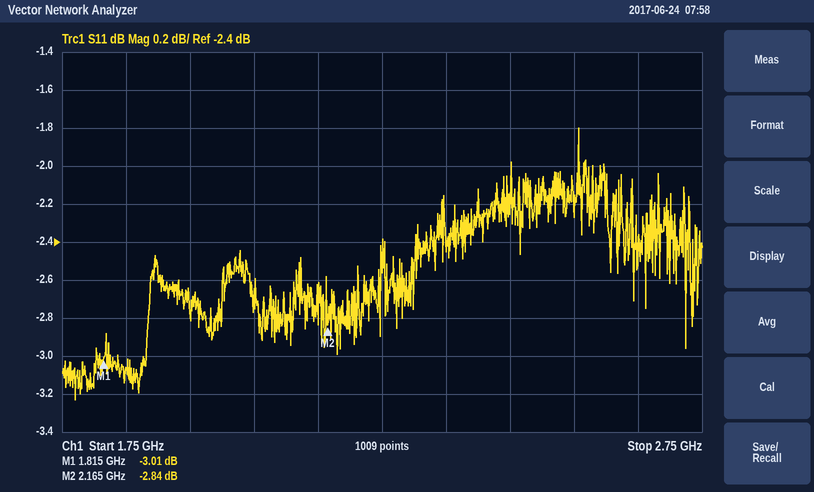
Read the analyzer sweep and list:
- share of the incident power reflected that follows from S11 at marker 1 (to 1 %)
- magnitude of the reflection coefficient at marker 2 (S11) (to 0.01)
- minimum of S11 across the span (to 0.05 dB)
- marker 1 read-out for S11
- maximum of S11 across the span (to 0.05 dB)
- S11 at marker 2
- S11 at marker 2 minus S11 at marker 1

50 %
0.72
-3.25 dB
-3.01 dB
-1.80 dB
-2.84 dB
0.17 dB
